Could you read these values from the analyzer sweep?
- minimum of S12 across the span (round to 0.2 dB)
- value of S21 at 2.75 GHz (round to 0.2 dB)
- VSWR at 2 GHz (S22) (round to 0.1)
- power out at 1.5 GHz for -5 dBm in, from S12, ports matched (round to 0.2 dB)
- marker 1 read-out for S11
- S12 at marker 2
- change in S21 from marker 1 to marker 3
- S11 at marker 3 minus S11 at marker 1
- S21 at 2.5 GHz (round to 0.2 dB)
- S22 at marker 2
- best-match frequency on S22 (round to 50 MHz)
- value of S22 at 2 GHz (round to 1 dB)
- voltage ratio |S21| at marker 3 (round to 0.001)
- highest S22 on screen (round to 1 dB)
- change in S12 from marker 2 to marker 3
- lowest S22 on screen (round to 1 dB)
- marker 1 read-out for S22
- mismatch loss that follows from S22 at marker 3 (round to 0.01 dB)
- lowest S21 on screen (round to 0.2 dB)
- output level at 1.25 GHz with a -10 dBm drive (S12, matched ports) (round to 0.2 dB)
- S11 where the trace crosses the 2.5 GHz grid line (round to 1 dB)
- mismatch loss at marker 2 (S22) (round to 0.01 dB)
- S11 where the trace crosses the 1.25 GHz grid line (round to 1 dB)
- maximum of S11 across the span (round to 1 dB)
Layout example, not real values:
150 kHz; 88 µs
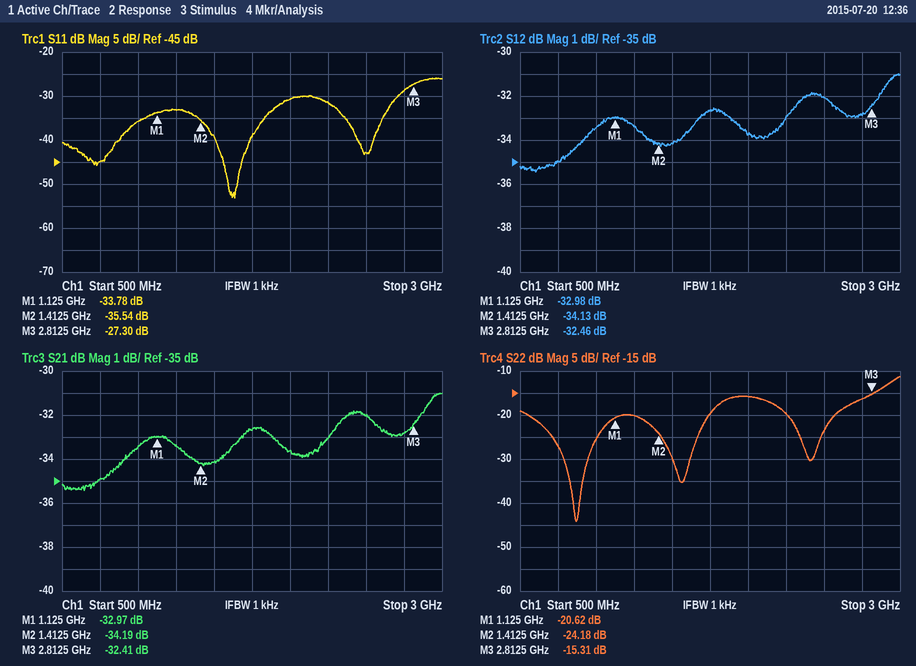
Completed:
-35.4 dB; -32.8 dB; 1.4; -39.2 dBm; -33.78 dB; -34.13 dB; 0.56 dB; 6.48 dB; -32.0 dB; -24.18 dB; 850 MHz; -16 dB; 0.024; -11 dB; 1.67 dB; -44 dB; -20.62 dB; 0.13 dB; -35.4 dB; -43.4 dBm; -43 dB; 0.02 dB; -33 dB; -26 dB
